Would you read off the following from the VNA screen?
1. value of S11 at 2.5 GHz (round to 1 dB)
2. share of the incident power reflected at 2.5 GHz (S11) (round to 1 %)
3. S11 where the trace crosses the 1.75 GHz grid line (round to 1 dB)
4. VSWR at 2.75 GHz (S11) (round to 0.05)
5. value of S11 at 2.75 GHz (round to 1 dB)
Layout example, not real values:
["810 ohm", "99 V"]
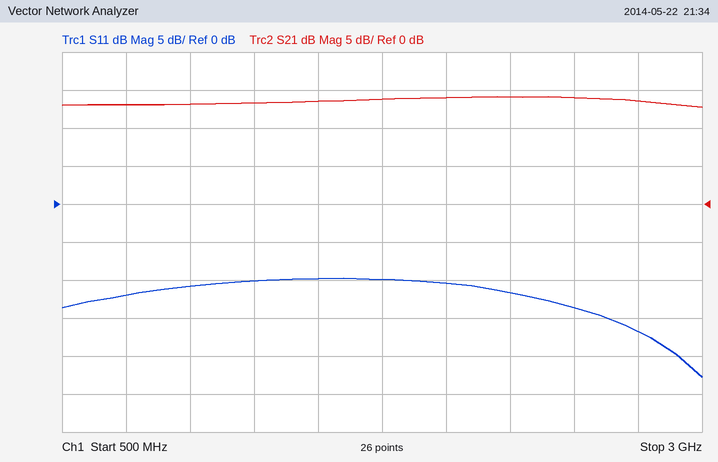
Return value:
["-14 dB", "4 %", "-10 dB", "1.35", "-17 dB"]
